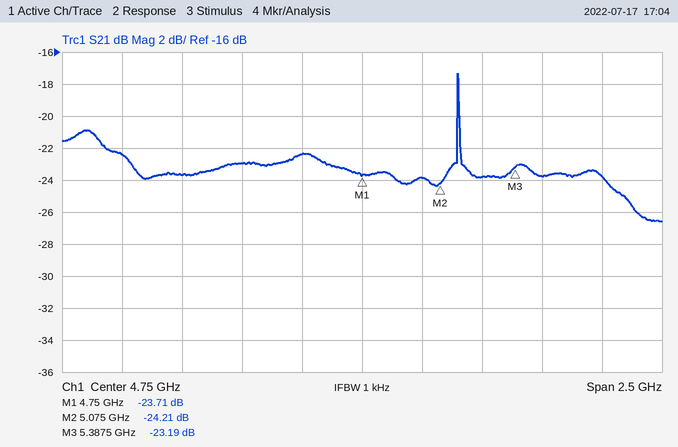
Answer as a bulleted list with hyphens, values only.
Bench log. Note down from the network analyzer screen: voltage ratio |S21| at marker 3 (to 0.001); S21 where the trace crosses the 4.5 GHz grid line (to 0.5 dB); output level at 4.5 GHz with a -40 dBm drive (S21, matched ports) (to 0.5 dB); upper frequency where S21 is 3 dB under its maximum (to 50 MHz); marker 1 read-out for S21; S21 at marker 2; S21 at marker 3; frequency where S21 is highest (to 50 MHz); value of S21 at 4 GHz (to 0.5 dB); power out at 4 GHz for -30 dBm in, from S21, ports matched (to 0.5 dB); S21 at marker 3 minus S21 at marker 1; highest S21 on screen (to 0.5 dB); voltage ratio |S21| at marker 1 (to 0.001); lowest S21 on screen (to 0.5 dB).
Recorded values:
- 0.069
- -22.5 dB
- -62.5 dBm
- 5.15 GHz
- -23.71 dB
- -24.21 dB
- -23.19 dB
- 5.15 GHz
- -23.5 dB
- -53.5 dBm
- 0.52 dB
- -17.5 dB
- 0.065
- -26.5 dB
